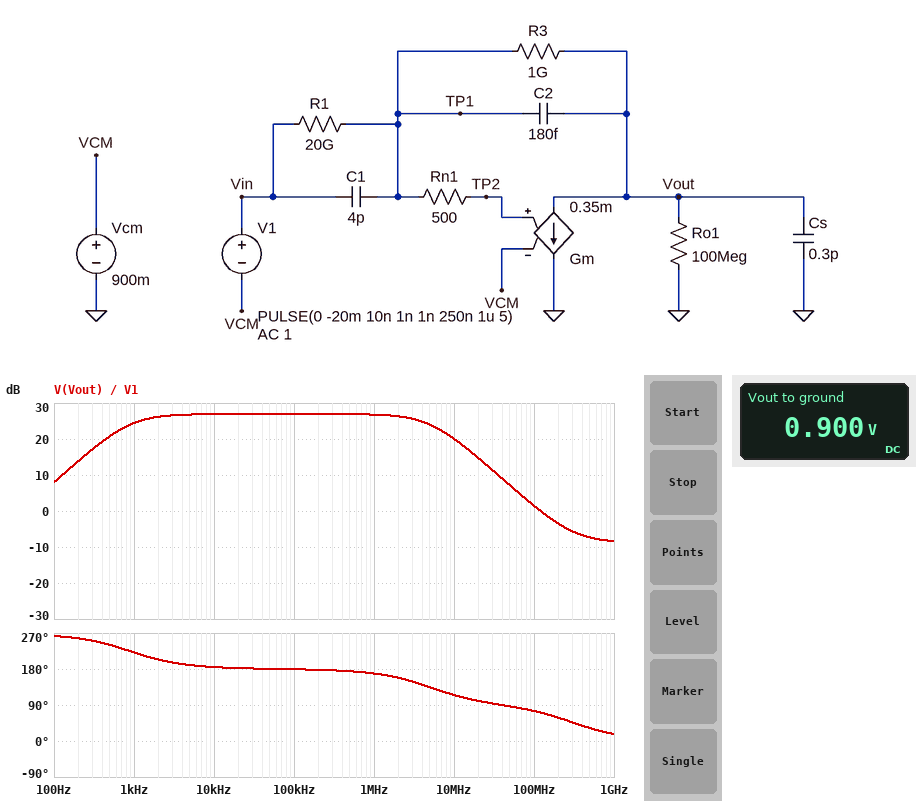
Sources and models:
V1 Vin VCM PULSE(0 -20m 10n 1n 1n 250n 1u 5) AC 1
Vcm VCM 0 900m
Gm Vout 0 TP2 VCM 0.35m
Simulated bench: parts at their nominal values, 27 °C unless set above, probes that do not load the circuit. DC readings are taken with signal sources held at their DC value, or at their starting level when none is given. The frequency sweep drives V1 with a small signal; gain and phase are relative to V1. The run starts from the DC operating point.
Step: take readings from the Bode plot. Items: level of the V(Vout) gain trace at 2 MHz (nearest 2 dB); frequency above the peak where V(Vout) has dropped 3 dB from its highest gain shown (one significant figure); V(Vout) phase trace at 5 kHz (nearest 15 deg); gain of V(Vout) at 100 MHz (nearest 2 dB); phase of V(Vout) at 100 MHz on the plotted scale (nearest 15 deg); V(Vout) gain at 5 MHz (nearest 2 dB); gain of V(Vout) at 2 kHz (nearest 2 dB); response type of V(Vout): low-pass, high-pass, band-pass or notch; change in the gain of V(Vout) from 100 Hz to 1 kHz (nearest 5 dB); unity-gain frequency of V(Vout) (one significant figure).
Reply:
26 dB
5 MHz
195 deg
2 dB
75 deg
24 dB
26 dB
band-pass
15 dB
100 MHz
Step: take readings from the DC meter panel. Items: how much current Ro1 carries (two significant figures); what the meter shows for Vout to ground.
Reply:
9.0 nA
0.900 V
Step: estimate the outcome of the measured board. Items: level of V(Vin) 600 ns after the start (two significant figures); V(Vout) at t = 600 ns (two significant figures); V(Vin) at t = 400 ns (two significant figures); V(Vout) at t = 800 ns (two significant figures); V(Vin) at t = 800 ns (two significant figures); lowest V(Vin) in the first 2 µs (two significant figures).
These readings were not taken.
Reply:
900 mV
900 mV
900 mV
900 mV
900 mV
880 mV
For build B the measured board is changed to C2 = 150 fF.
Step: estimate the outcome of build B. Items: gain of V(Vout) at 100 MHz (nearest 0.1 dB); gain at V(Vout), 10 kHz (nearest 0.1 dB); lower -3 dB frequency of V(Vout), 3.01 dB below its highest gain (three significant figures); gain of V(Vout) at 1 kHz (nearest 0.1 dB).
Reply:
1.9 dB
28.5 dB
1.06 kHz
25.2 dB
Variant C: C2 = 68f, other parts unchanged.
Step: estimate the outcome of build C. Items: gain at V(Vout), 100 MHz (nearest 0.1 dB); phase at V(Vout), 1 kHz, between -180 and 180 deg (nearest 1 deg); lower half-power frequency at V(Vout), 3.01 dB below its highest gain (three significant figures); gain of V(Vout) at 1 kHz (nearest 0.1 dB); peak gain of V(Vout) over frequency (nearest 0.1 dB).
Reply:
3.5 dB
-113 deg
2.33 kHz
27.3 dB
35.4 dB
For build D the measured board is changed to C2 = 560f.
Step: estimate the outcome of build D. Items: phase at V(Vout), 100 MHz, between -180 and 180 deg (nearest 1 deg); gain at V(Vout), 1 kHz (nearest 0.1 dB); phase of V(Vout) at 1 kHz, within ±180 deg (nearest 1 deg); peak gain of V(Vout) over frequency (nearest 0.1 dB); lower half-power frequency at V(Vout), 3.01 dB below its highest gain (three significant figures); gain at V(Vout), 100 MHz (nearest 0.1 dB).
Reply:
50 deg
16.7 dB
-164 deg
17.1 dB
284 Hz
-1.2 dB
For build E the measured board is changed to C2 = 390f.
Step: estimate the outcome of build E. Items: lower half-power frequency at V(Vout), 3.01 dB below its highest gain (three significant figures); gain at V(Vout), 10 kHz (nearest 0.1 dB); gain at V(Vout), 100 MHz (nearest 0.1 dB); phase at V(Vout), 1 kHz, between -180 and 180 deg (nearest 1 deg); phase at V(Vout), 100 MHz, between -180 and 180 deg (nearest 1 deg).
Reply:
408 Hz
20.2 dB
-0.5 dB
-158 deg
59 deg
